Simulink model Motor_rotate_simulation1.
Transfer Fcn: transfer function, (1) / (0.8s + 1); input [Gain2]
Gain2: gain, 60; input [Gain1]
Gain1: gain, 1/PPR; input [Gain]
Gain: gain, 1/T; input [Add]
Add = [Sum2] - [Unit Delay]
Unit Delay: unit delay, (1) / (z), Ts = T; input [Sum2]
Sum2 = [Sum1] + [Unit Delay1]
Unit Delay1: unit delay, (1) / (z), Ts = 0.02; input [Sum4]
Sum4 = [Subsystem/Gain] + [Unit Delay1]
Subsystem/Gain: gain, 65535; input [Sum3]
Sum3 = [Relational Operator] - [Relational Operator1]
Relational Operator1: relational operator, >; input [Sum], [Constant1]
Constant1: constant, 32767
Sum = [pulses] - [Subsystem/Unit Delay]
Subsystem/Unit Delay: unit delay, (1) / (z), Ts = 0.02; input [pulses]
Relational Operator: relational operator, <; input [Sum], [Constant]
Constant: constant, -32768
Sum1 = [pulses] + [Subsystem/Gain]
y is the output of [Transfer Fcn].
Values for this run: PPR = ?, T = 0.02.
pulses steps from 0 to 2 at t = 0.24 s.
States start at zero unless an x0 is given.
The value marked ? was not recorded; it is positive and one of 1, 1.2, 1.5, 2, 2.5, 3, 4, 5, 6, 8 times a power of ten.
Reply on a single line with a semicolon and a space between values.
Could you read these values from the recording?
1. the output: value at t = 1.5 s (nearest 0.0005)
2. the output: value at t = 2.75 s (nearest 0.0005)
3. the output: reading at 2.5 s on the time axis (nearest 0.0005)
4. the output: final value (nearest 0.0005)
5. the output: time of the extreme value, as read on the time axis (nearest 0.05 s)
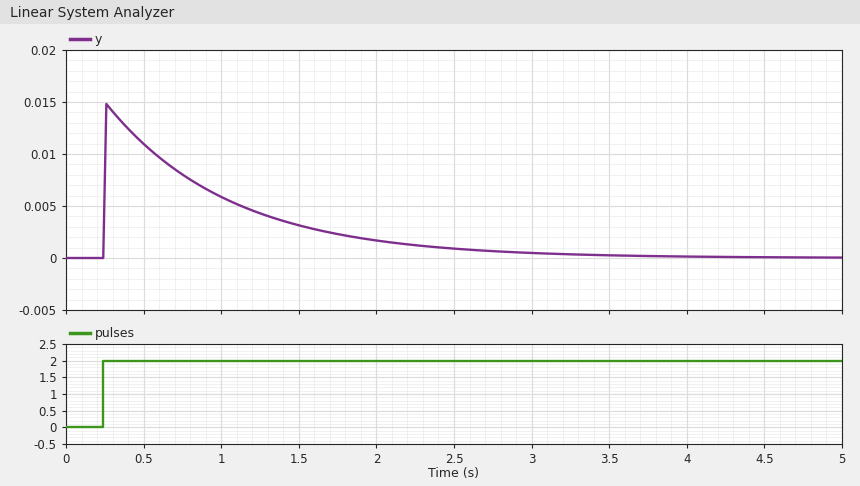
0.0030; 0.0005; 0.0010; 0.0000; 0.25 s
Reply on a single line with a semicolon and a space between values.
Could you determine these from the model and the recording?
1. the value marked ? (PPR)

10000
